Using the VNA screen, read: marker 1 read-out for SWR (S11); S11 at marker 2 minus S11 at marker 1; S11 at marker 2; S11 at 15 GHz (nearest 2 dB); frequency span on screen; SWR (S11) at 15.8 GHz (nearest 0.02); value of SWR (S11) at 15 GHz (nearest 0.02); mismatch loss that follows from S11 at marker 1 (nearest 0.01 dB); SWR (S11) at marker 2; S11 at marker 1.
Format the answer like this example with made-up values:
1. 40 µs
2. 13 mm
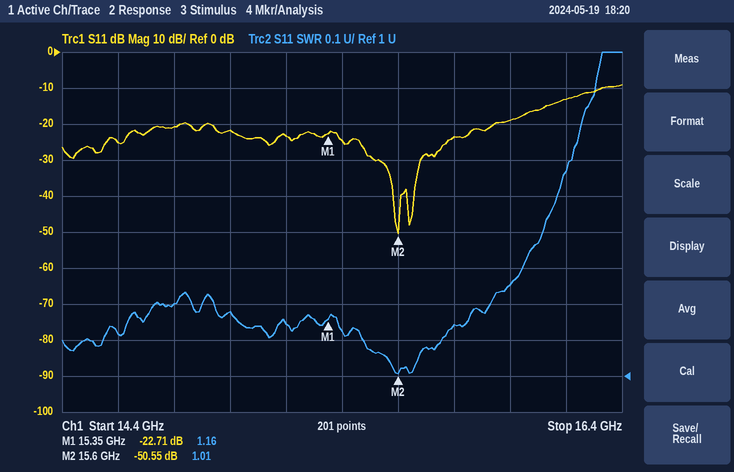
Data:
1. 1.16
2. -27.84 dB
3. -50.55 dB
4. -22 dB
5. 2 GHz
6. 1.14
7. 1.18
8. 0.02 dB
9. 1.01
10. -22.71 dB
